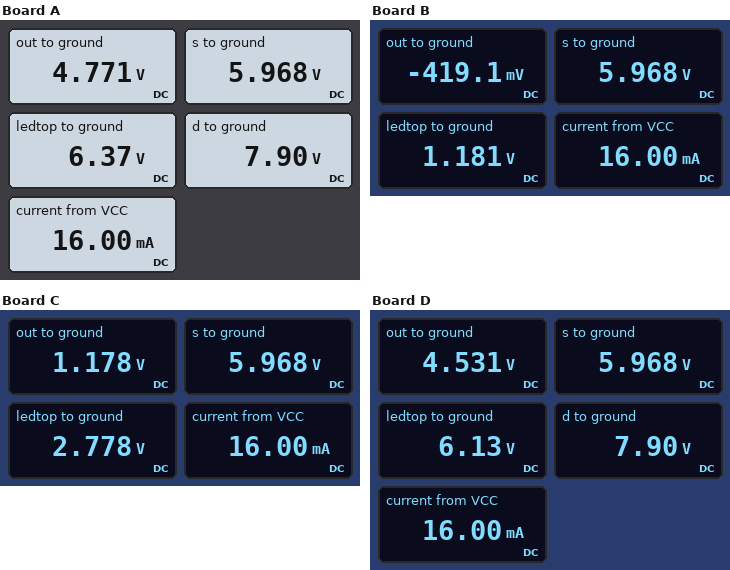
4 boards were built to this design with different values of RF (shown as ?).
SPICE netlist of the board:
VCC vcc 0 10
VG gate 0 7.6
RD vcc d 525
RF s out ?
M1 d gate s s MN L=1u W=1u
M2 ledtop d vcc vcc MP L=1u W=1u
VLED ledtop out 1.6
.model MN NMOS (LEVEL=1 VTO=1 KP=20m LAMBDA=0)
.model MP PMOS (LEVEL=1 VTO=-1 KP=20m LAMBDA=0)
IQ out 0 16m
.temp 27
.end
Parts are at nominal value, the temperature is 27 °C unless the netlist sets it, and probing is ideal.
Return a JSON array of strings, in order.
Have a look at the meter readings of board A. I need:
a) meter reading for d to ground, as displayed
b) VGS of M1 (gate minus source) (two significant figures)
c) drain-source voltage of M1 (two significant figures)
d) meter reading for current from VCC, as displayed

["7.90 V", "1.6 V", "1.9 V", "16.00 mA"]
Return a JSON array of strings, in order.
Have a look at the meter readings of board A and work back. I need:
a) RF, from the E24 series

["300 Ω"]
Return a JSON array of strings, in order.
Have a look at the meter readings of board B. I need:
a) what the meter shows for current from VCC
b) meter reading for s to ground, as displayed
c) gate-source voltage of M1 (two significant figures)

["16.00 mA", "5.968 V", "1.6 V"]
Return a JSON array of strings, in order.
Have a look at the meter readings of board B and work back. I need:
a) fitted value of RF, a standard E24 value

["1.6 kΩ"]
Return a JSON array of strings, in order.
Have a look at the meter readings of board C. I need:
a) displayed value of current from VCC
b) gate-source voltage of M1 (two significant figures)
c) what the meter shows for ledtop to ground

["16.00 mA", "1.6 V", "2.778 V"]
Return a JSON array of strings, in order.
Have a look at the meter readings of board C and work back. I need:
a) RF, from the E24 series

["1.2 kΩ"]
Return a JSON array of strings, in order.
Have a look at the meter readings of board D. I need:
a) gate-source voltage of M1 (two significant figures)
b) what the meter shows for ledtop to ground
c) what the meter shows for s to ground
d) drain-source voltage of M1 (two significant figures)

["1.6 V", "6.13 V", "5.968 V", "1.9 V"]
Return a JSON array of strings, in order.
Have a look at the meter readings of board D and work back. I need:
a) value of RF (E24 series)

["360 Ω"]
